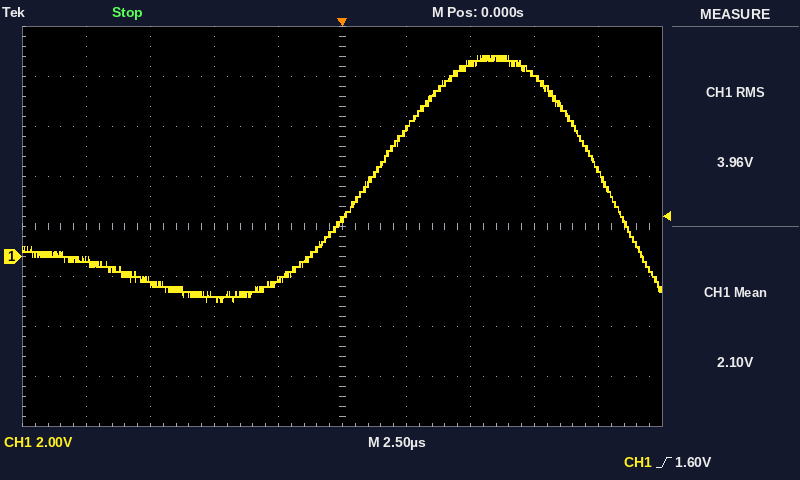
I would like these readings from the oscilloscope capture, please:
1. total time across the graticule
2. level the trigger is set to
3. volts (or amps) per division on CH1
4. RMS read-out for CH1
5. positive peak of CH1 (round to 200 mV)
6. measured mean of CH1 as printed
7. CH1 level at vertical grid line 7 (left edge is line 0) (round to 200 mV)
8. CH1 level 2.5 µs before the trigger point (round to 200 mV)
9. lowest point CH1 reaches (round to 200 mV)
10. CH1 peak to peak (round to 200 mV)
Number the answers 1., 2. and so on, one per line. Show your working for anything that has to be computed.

1. 25 µs
2. 1.60 V
3. 2 V
4. 3.96 V
5. 8.0 V
6. 2.10 V
7. 7.8 V
8. -1.0 V
9. -1.8 V
10. 8.0 V − (-1.8 V) = 9.8 V
